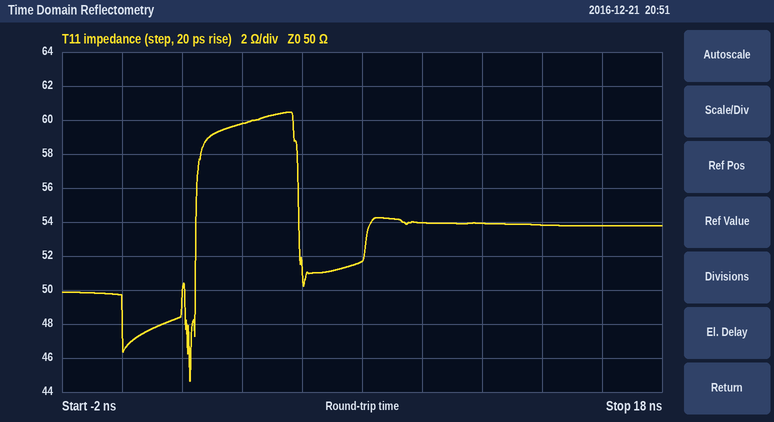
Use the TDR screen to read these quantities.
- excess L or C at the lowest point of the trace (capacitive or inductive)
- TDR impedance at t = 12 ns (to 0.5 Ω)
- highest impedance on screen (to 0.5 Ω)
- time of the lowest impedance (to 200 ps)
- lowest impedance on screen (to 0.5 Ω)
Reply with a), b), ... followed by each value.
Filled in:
a) capacitive
b) 54.0 Ω
c) 60.5 Ω
d) 2.2 ns
e) 44.5 Ω
